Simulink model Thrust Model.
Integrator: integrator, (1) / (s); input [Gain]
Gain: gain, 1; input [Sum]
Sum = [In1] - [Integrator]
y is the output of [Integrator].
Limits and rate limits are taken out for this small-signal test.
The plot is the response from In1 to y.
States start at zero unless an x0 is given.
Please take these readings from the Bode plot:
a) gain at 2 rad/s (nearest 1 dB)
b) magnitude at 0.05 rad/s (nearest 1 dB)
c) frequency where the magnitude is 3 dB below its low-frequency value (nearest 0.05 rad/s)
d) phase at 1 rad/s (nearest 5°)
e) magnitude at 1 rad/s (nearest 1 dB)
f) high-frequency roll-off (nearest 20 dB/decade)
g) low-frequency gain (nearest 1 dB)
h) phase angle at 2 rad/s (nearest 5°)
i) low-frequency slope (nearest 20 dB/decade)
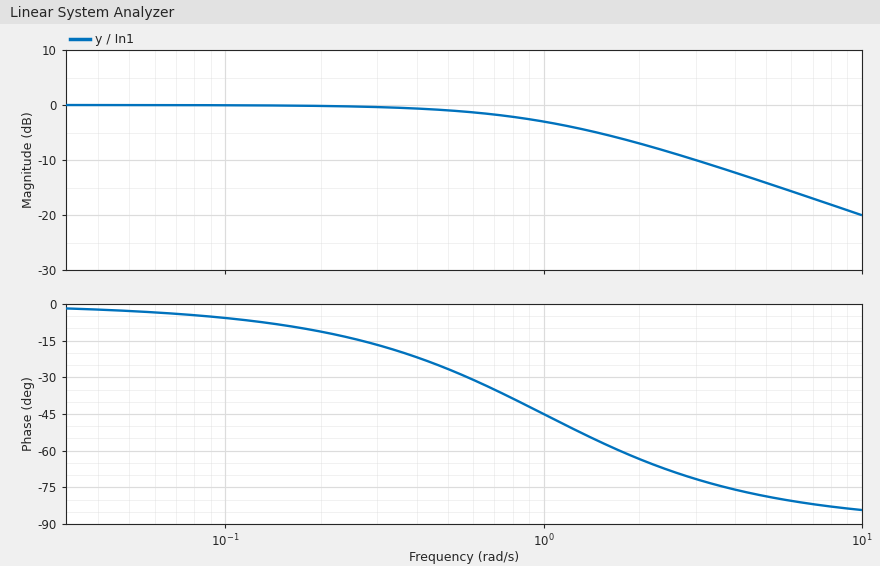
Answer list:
-7 dB
0 dB
1.00 rad/s
-45°
-3 dB
-20 dB/decade
0 dB
-65°
0 dB/decade
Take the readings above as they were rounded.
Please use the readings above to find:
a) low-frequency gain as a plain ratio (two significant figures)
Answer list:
1.0
